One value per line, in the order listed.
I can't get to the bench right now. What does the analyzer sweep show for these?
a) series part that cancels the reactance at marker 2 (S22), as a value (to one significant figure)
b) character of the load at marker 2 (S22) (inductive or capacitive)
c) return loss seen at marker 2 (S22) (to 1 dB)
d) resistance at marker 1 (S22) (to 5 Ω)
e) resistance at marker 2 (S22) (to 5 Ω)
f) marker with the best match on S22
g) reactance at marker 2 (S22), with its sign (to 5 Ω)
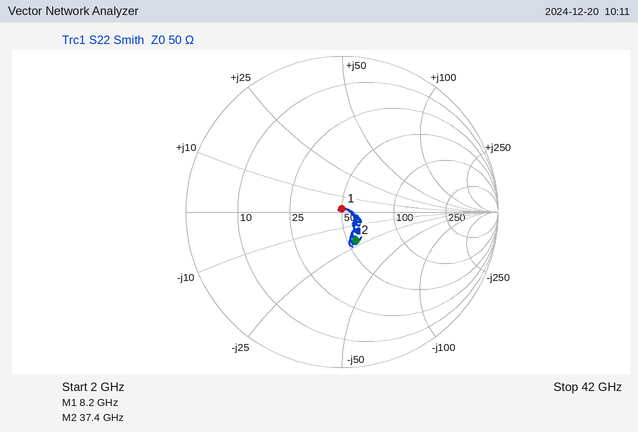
90 pH
capacitive
14 dB
50 Ω
55 Ω
marker 1
-20 Ω
